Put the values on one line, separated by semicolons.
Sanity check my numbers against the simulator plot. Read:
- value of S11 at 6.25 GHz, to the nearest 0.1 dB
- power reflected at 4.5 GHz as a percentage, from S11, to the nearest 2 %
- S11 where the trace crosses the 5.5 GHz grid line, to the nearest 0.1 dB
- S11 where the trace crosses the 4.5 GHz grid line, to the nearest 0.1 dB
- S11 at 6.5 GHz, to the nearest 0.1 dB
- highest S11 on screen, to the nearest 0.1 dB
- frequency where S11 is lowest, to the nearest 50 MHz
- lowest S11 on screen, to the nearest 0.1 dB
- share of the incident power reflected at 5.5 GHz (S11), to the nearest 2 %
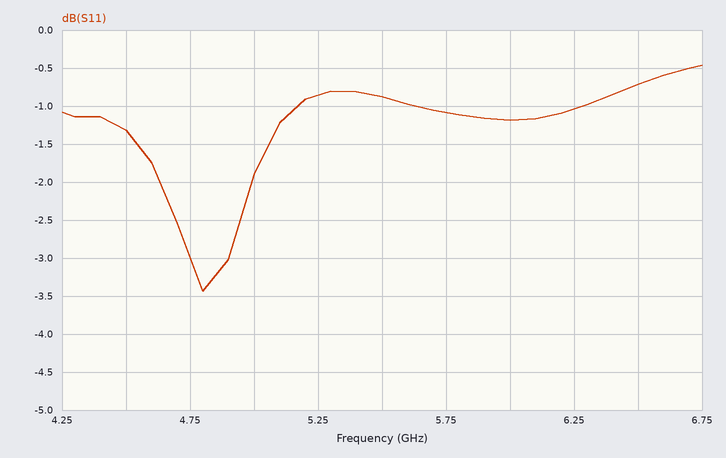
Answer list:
-1.0 dB; 74 %; -0.9 dB; -1.3 dB; -0.7 dB; -0.5 dB; 4.80 GHz; -3.4 dB; 82 %
